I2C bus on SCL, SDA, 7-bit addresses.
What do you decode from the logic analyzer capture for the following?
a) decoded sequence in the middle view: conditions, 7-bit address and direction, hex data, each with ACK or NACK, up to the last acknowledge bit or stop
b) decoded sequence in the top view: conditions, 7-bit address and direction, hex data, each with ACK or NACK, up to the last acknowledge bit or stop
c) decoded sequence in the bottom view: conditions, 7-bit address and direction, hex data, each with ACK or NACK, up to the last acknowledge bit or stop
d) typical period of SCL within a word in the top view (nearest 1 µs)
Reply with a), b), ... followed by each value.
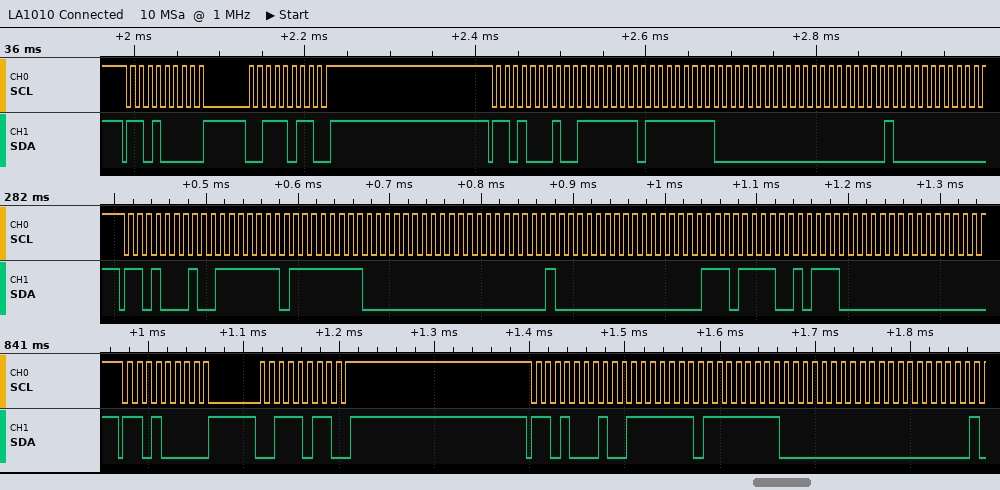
a) start, address 68 read ACK, 7F ACK, FF ACK, 00 ACK, 00 ACK, 40 ACK, 00 ACK, EF ACK, 5C ACK, 00 ACK
b) start, address 68 write ACK, 3B ACK, stop, start, address 68 read ACK, 7F ACK, FF ACK, 00 ACK, 00 ACK, 40 ACK
c) start, address 68 write ACK, 3B ACK, stop, start, address 68 read ACK, 7F ACK, FF ACK, 00 ACK, 00 ACK
d) 10 µs
